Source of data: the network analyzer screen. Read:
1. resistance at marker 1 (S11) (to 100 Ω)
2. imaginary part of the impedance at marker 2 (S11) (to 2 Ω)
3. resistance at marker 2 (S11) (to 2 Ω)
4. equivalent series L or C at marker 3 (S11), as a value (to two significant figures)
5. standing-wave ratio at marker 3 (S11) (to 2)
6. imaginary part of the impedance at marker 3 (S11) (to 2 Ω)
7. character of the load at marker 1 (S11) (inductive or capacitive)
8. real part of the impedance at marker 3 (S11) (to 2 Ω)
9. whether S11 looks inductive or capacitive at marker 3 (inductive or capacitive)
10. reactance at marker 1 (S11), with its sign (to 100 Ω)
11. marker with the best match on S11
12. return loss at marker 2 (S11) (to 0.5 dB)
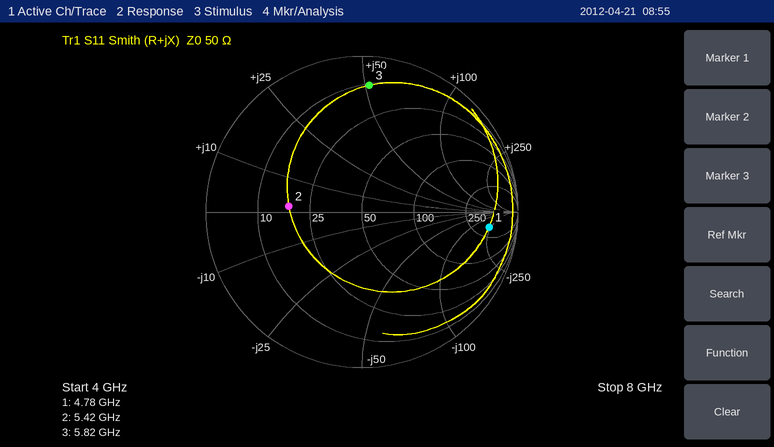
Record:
400 Ω
+2 Ω
18 Ω
1.4 nH
10
+52 Ω
capacitive
10 Ω
inductive
-200 Ω
marker 2
6.5 dB
